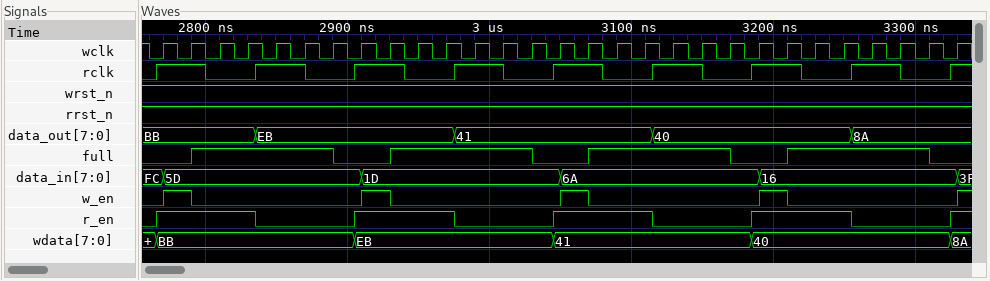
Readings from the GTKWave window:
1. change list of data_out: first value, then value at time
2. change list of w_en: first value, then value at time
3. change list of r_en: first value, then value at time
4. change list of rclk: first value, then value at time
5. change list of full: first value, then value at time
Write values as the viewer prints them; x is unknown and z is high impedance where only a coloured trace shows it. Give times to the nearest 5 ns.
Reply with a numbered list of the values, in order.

1. BB, EB at 2835 ns, 41 at 2975 ns, 40 at 3115 ns, 8A at 3255 ns
2. 0, 1 at 2770 ns, 0 at 2790 ns, 1 at 2910 ns, 0 at 2930 ns, 1 at 3050 ns, 0 at 3070 ns, 1 at 3190 ns, 0 at 3210 ns, 1 at 3330 ns
3. 0, 1 at 2765 ns, 0 at 2835 ns, 1 at 2905 ns, 0 at 2975 ns, 1 at 3045 ns, 0 at 3115 ns, 1 at 3185 ns, 0 at 3255 ns, 1 at 3325 ns
4. 0, 1 at 2765 ns, 0 at 2800 ns, 1 at 2835 ns, 0 at 2870 ns, 1 at 2905 ns, 0 at 2940 ns, 1 at 2975 ns, 0 at 3010 ns, 1 at 3045 ns, 0 at 3080 ns, 1 at 3115 ns, 0 at 3150 ns, 1 at 3185 ns, 0 at 3220 ns, 1 at 3255 ns, 0 at 3290 ns, 1 at 3325 ns
5. 0, 1 at 2790 ns, 0 at 2890 ns, 1 at 2930 ns, 0 at 3030 ns, 1 at 3070 ns, 0 at 3170 ns, 1 at 3210 ns, 0 at 3310 ns
